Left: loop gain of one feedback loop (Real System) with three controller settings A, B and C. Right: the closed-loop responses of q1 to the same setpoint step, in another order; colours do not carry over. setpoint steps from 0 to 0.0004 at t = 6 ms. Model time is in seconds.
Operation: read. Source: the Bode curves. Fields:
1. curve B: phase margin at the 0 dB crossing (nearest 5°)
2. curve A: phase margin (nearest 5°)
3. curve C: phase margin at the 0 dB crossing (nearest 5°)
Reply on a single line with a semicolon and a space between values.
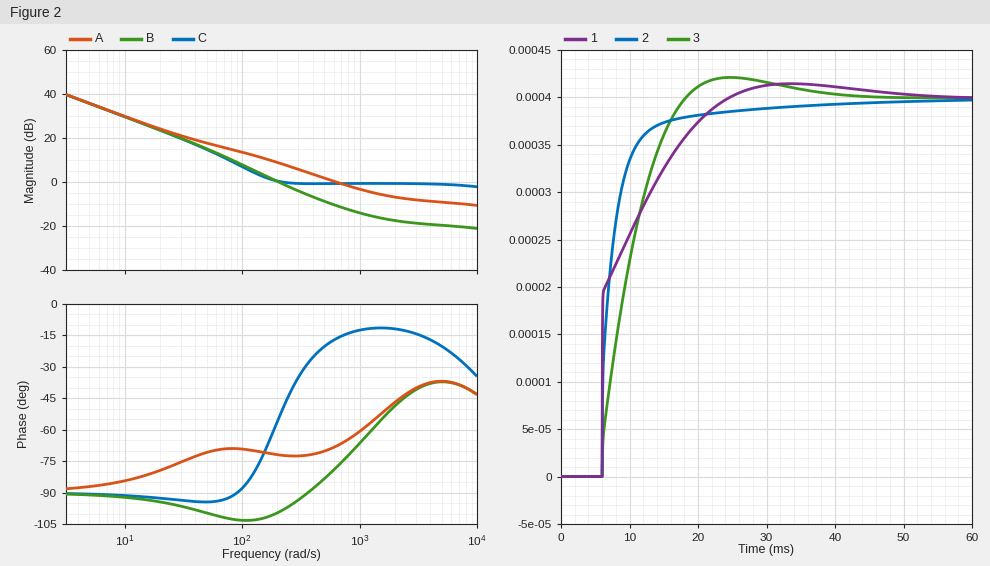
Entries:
80°; 110°; 130°
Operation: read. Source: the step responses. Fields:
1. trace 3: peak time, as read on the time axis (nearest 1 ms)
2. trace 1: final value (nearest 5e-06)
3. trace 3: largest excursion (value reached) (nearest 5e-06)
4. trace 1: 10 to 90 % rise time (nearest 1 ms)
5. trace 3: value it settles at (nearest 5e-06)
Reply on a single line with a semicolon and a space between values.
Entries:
25 ms; 0.000400; 0.000420; 12 ms; 0.000400
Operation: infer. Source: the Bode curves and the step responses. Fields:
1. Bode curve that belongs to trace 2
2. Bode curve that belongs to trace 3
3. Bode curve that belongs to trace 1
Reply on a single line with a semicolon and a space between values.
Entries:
A; B; C
